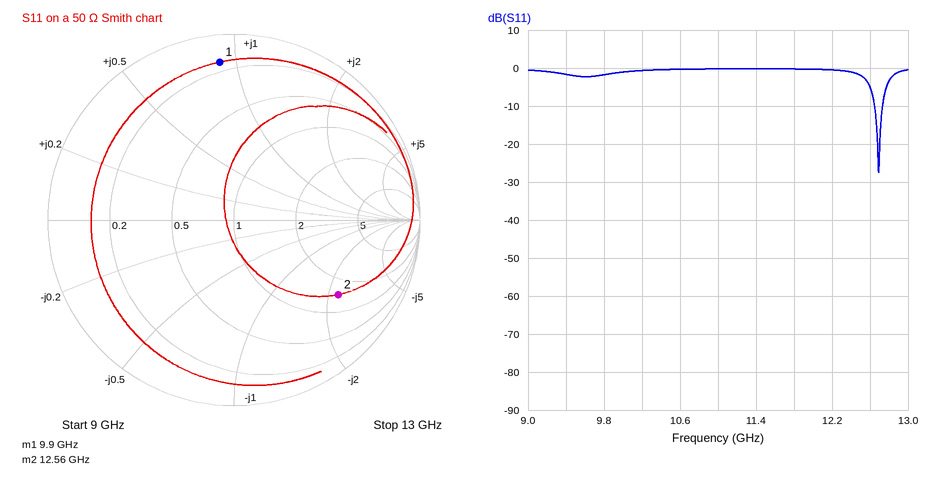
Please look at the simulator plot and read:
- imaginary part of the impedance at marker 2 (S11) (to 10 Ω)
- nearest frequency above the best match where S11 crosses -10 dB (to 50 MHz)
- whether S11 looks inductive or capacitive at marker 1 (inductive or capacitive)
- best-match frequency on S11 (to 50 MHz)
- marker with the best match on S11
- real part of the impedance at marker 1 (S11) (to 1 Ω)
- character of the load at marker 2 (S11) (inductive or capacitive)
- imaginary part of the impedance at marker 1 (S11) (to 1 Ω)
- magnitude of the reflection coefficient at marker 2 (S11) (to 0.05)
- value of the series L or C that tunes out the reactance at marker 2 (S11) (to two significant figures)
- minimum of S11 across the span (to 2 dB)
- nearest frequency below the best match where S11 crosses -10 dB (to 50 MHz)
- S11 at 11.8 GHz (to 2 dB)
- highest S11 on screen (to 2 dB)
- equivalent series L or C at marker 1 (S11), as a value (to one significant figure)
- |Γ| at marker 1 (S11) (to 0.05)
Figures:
-110 Ω
12.75 GHz
inductive
12.70 GHz
marker 2
7 Ω
capacitive
+45 Ω
0.70
1.4 nH
-28 dB
12.65 GHz
0 dB
0 dB
700 pH
0.85
